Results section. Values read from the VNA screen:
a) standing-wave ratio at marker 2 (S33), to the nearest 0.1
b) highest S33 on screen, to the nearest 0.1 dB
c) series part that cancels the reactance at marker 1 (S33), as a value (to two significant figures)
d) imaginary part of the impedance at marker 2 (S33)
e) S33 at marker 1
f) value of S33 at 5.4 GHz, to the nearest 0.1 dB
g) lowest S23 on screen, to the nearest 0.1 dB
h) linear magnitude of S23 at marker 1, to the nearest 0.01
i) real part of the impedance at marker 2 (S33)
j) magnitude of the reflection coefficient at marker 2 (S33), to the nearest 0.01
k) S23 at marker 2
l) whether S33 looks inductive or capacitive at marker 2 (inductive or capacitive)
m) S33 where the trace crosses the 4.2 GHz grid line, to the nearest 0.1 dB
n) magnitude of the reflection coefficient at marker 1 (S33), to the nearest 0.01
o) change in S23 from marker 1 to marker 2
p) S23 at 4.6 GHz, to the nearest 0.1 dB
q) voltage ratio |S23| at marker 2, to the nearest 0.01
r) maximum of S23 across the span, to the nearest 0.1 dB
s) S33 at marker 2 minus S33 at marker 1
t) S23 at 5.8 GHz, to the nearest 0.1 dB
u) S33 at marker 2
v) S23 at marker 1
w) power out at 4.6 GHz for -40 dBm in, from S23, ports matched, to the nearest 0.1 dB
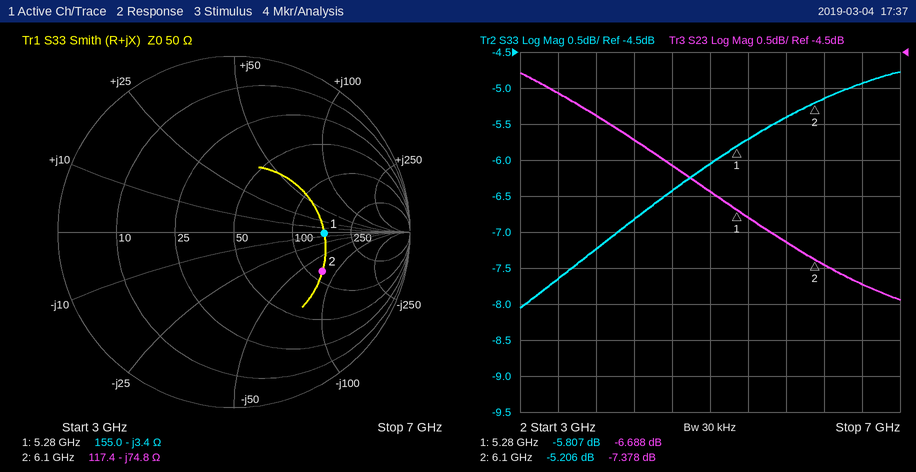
3.4
-4.8 dB
100 pH
-74.8 Ω
-5.807 dB
-5.7 dB
-7.9 dB
0.46
117.4 Ω
0.55
-7.378 dB
capacitive
-6.8 dB
0.51
-0.690 dB
-6.1 dB
0.43
-4.8 dB
0.601 dB
-7.1 dB
-5.206 dB
-6.688 dB
-46.1 dBm
